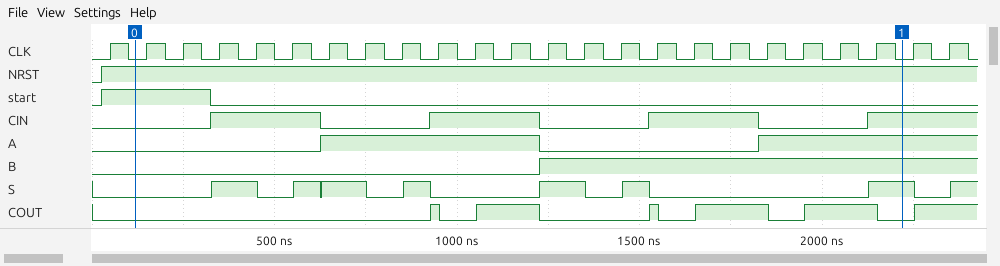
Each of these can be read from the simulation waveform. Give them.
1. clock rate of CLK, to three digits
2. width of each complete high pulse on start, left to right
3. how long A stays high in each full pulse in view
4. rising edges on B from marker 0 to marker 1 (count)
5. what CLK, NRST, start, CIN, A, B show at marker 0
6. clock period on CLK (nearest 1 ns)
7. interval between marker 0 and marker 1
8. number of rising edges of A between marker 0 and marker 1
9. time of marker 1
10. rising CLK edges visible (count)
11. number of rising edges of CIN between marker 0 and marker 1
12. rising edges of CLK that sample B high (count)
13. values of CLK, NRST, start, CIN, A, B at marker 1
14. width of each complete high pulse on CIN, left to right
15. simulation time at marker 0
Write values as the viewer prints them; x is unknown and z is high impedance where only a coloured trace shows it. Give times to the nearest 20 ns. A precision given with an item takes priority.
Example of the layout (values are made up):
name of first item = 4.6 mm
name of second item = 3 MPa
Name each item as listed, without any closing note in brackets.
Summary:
clock rate of CLK, to three digits = 10.0 MHz
width of each complete high pulse on start, left to right = 300 ns
how long A stays high in each full pulse in view = 600 ns
rising edges on B from marker 0 to marker 1 = 1
what CLK, NRST, start, CIN, A, B show at marker 0 = CLK=0, NRST=1, start=1, CIN=0, A=0, B=0
clock period on CLK = 100 ns
interval between marker 0 and marker 1 = 2100 ns
number of rising edges of A between marker 0 and marker 1 = 2
time of marker 1 = 2220 ns
rising CLK edges visible = 24
number of rising edges of CIN between marker 0 and marker 1 = 4
rising edges of CLK that sample B high = 12
values of CLK, NRST, start, CIN, A, B at marker 1 = CLK=0, NRST=1, start=0, CIN=1, A=1, B=1
width of each complete high pulse on CIN, left to right = 300 ns, 300 ns, 300 ns
simulation time at marker 0 = 120 ns
